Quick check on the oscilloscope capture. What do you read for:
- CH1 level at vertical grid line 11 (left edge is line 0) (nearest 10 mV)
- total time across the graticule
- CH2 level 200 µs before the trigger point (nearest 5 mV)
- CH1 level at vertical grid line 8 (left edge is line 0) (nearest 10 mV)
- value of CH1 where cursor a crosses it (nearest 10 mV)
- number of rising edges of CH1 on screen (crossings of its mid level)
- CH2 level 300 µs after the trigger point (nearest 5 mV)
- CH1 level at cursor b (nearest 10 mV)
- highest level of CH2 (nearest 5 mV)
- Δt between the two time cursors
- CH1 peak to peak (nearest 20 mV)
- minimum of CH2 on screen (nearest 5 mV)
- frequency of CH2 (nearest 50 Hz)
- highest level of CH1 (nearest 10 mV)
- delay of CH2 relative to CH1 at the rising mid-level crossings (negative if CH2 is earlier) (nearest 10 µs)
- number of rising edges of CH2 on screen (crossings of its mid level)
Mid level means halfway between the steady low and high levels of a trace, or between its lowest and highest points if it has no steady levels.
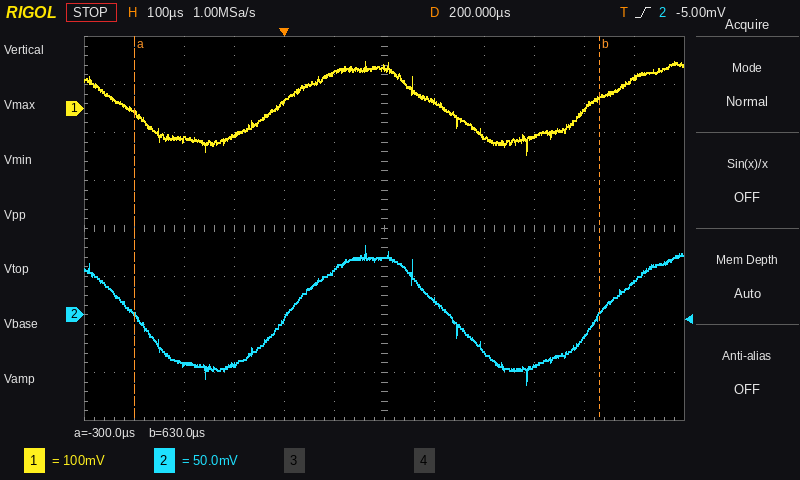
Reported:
60 mV
1.2 ms
-50 mV
-60 mV
-10 mV
2
15 mV
20 mV
70 mV
930 µs
200 mV
-70 mV
1.60 kHz
100 mV
+20 µs
2
